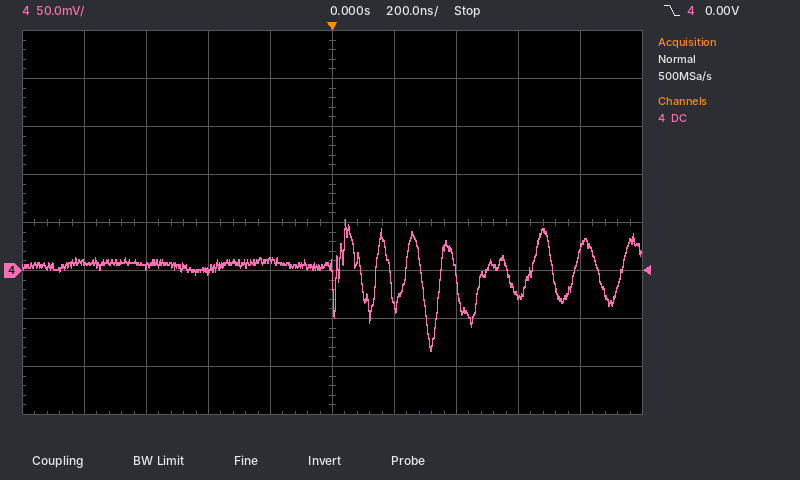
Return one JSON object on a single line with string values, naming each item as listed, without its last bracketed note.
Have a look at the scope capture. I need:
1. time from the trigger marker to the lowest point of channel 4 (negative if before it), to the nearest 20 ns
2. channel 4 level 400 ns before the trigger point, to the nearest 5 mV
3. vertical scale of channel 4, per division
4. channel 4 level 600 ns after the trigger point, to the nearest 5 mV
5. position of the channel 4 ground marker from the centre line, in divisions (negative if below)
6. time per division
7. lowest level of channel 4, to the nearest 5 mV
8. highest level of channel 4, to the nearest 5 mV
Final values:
{"time from the trigger marker to the lowest point of channel 4 (negative if before it), to the nearest 20 ns": "+320 ns", "channel 4 level 400 ns before the trigger point, to the nearest 5 mV": "0 mV", "vertical scale of channel 4, per division": "50 mV", "channel 4 level 600 ns after the trigger point, to the nearest 5 mV": "-25 mV", "position of the channel 4 ground marker from the centre line, in divisions": "-1.0 div", "time per division": "200 ns", "lowest level of channel 4, to the nearest 5 mV": "-85 mV", "highest level of channel 4, to the nearest 5 mV": "55 mV"}
